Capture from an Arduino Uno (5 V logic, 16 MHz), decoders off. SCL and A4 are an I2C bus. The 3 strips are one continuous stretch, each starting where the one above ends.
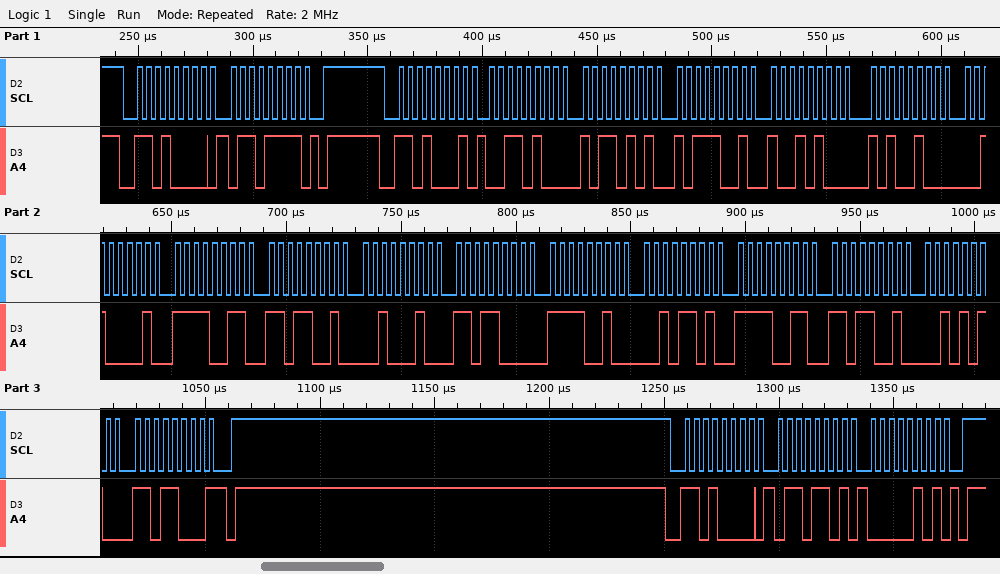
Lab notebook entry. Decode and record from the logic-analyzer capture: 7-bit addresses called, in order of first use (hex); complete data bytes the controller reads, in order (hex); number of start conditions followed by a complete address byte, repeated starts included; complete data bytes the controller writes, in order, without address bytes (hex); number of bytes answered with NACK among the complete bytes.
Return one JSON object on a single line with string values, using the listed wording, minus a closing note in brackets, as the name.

{"7-bit addresses called, in order of first use": "0x68", "complete data bytes the controller reads, in order": "34 B5 B9 94 A4 21 F3 D9 22 D8 F2 2D F3 D9 2A D8", "number of start conditions followed by a complete address byte, repeated starts included": "3", "complete data bytes the controller writes, in order, without address bytes": "6F 6D 05", "number of bytes answered with NACK among the complete bytes": "1"}
